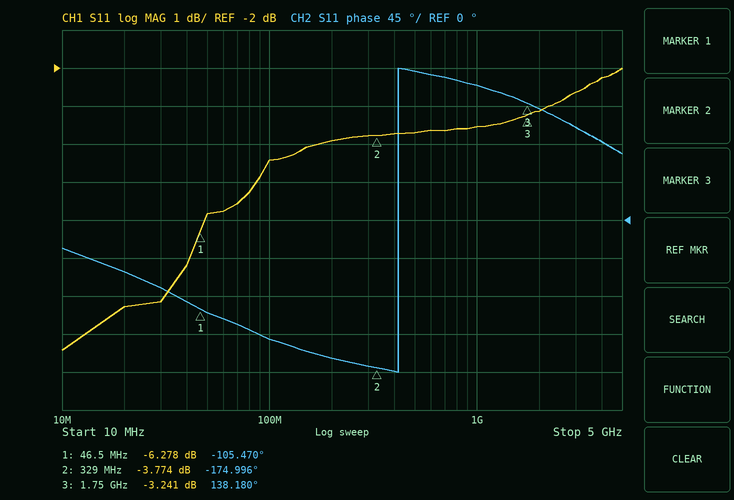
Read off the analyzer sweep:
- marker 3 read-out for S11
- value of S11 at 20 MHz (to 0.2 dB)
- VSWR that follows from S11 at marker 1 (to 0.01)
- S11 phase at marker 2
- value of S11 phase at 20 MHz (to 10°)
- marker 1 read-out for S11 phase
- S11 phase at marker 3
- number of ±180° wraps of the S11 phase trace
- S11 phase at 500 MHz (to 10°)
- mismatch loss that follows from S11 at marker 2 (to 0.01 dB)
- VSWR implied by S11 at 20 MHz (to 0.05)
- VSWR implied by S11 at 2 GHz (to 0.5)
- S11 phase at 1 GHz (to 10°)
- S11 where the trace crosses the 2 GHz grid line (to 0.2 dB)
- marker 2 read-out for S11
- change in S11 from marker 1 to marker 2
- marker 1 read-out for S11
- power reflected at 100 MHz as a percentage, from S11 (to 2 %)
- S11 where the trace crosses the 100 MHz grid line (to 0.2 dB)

-3.241 dB
-8.2 dB
2.89
-174.996°
-60°
-105.470°
138.180°
1
180°
2.36 dB
2.25
5.5
160°
-3.2 dB
-3.774 dB
2.504 dB
-6.278 dB
36 %
-4.4 dB
